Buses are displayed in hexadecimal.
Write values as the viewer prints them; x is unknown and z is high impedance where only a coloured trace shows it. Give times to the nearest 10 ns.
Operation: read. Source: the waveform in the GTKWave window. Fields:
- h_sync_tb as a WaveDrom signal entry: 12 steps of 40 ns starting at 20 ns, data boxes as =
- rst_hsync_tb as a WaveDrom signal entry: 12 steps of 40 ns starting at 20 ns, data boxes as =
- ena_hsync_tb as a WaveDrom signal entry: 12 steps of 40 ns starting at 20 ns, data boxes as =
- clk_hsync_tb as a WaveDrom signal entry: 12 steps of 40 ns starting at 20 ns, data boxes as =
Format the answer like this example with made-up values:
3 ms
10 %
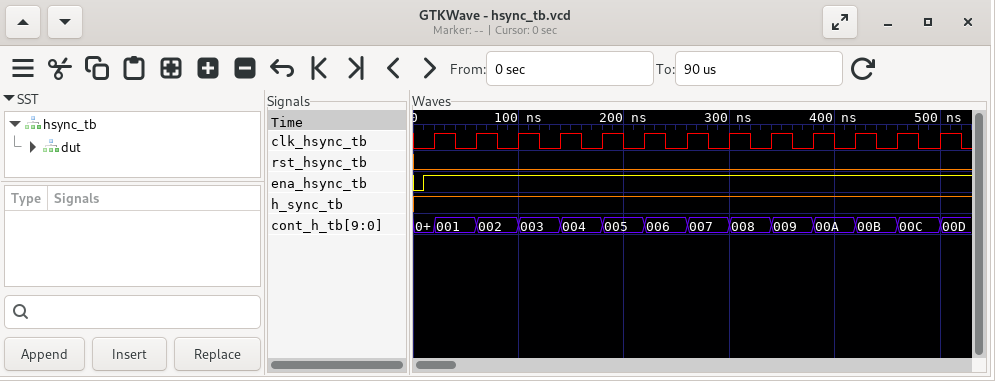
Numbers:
{name: 'h_sync_tb', wave: '1...........'}
{name: 'rst_hsync_tb', wave: '0...........'}
{name: 'ena_hsync_tb', wave: '1...........'}
{name: 'clk_hsync_tb', wave: 'p...........'}
